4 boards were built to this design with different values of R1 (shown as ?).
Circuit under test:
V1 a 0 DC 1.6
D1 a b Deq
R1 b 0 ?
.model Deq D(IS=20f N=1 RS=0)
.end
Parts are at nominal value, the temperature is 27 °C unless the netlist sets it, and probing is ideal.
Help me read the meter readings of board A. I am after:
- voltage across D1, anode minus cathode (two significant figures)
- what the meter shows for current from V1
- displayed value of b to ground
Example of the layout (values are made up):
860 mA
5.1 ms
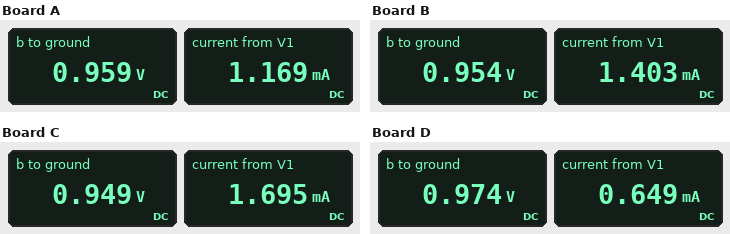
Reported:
640 mV
1.169 mA
0.959 V
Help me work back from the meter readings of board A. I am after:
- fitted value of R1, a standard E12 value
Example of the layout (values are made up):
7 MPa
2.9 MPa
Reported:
820 Ω
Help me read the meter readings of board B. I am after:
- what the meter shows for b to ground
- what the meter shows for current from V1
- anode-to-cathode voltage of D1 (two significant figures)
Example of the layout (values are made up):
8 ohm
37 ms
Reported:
0.954 V
1.403 mA
650 mV
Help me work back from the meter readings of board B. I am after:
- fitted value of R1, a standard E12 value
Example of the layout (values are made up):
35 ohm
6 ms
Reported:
680 Ω
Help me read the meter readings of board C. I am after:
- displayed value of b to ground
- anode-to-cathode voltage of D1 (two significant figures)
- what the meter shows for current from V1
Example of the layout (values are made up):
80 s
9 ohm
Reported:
0.949 V
650 mV
1.695 mA
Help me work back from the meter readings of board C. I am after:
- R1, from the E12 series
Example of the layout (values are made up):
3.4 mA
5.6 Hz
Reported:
560 Ω
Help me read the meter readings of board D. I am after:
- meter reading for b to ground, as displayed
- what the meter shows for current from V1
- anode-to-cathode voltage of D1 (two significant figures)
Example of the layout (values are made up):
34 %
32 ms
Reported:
0.974 V
0.649 mA
630 mV
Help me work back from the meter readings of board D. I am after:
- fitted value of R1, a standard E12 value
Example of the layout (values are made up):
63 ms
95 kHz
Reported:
1.5 kΩ
